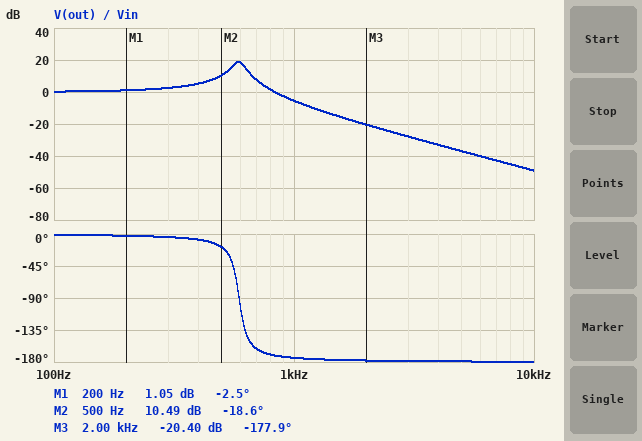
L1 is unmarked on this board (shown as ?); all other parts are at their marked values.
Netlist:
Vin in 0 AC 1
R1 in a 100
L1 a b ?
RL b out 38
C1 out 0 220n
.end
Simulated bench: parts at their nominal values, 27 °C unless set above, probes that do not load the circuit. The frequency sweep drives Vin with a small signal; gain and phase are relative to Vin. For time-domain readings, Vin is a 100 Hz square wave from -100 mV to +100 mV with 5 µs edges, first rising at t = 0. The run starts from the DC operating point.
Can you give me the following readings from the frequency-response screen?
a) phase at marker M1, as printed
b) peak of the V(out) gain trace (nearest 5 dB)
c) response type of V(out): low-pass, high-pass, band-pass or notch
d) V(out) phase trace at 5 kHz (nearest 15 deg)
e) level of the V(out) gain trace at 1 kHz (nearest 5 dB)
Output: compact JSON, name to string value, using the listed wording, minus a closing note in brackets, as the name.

{"phase at marker M1, as printed": "-2.5 deg", "peak of the V(out) gain trace": "20 dB", "response type of V(out): low-pass, high-pass, band-pass or notch": "low-pass", "V(out) phase trace at 5 kHz": "-180 deg", "level of the V(out) gain trace at 1 kHz": "-5 dB"}
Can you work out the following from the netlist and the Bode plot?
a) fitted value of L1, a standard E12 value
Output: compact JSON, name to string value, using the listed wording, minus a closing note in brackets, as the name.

{"fitted value of L1, a standard E12 value": "330 mH"}
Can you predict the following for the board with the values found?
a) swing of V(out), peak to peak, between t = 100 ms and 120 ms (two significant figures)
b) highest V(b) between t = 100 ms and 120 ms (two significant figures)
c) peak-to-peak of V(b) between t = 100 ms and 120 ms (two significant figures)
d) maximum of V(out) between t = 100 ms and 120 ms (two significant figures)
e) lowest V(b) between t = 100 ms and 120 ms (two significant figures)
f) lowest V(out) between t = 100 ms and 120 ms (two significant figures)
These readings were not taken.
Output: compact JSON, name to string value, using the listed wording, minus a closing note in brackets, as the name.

{"swing of V(out), peak to peak, between t = 100 ms and 120 ms": "450 mV", "highest V(b) between t = 100 ms and 120 ms": "230 mV", "peak-to-peak of V(b) between t = 100 ms and 120 ms": "450 mV", "maximum of V(out) between t = 100 ms and 120 ms": "230 mV", "lowest V(b) between t = 100 ms and 120 ms": "-230 mV", "lowest V(out) between t = 100 ms and 120 ms": "-230 mV"}
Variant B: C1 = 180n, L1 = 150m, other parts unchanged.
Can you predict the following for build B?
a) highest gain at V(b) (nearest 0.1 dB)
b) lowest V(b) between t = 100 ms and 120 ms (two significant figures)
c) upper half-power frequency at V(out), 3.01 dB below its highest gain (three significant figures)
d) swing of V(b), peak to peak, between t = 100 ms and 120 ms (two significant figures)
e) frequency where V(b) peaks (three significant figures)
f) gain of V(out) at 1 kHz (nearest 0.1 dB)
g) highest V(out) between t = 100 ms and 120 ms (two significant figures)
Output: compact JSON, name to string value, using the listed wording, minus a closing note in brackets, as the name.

{"highest gain at V(b)": "16.4 dB", "lowest V(b) between t = 100 ms and 120 ms": "-250 mV", "upper half-power frequency at V(out), 3.01 dB below its highest gain": "1.03 kHz", "swing of V(b), peak to peak, between t = 100 ms and 120 ms": "500 mV", "frequency where V(b) peaks": "963 Hz", "gain of V(out) at 1 kHz": "15.4 dB", "highest V(out) between t = 100 ms and 120 ms": "250 mV"}
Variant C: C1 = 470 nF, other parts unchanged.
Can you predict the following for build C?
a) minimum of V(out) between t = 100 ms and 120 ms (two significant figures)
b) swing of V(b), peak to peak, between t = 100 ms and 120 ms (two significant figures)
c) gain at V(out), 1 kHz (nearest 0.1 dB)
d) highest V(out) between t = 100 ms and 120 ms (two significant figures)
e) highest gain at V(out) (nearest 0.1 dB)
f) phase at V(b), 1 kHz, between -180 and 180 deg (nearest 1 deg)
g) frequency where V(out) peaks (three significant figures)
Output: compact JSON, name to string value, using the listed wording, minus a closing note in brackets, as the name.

{"minimum of V(out) between t = 100 ms and 120 ms": "-210 mV", "swing of V(b), peak to peak, between t = 100 ms and 120 ms": "430 mV", "gain at V(out), 1 kHz": "-14.2 dB", "highest V(out) between t = 100 ms and 120 ms": "210 mV", "highest gain at V(out)": "15.7 dB", "phase at V(b), 1 kHz, between -180 and 180 deg": "-169 deg", "frequency where V(out) peaks": "401 Hz"}
